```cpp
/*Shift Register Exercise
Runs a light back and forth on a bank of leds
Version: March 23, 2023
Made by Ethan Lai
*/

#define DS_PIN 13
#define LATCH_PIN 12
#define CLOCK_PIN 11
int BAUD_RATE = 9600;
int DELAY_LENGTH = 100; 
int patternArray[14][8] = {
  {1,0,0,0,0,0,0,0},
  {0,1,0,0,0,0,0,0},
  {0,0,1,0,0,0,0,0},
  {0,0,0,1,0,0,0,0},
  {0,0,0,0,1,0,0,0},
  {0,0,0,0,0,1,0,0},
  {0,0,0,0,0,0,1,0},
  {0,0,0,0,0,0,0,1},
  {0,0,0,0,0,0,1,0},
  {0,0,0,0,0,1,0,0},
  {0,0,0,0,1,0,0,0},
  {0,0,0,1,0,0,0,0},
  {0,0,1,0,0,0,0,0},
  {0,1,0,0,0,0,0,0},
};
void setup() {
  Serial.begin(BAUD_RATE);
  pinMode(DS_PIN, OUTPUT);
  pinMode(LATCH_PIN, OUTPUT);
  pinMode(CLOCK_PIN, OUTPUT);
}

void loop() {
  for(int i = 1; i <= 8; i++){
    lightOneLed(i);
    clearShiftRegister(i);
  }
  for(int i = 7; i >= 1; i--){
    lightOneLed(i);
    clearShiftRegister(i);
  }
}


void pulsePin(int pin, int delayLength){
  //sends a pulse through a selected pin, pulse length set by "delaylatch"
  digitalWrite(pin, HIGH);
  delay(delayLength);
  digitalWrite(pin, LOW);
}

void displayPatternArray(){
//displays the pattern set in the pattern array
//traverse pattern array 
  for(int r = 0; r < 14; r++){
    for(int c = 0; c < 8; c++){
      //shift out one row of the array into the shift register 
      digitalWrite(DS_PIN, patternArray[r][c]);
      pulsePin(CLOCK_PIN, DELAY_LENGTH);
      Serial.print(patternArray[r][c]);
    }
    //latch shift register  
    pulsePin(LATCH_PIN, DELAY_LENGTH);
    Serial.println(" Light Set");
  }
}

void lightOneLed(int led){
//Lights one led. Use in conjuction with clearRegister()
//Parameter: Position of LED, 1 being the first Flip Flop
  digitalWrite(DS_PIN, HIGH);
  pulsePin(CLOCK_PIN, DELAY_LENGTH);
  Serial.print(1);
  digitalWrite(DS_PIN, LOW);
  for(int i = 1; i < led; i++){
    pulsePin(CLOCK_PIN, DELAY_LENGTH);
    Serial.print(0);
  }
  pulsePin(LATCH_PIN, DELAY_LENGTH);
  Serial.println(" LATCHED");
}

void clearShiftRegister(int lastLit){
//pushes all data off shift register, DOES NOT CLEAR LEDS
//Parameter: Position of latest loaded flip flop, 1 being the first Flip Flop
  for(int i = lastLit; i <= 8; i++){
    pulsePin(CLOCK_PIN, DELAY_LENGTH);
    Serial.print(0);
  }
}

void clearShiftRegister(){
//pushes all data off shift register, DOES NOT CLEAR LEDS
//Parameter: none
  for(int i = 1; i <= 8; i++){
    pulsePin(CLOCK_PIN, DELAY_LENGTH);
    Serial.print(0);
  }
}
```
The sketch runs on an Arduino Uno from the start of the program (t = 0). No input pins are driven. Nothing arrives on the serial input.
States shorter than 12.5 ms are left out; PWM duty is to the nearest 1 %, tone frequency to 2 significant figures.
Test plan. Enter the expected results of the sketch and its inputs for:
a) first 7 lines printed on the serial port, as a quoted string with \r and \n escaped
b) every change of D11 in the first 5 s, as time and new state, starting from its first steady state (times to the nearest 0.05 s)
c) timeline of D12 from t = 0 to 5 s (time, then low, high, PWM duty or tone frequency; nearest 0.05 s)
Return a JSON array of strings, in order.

["\"1 LATCHED\\r\\n0000000010 LATCHED\\r\\n0000000100 LATCHED\\r\\n0000001000 LATCHED\\r\\n0000010000 LATCHED\\r\\n0000100000 LATCHED\\r\\n0001000000 LATCHED\\r\\n\"", "0 s high; 0.1 s low; 0.2 s high; 1.2 s low; 1.3 s high; 2.3 s low; 2.4 s high; 3.4 s low; 3.5 s high; 4.5 s low; 4.6 s high", "0 s low; 0.1 s high; 0.2 s low; 1.2 s high; 1.3 s low; 2.3 s high; 2.4 s low; 3.4 s high; 3.5 s low; 4.5 s high; 4.6 s low"]
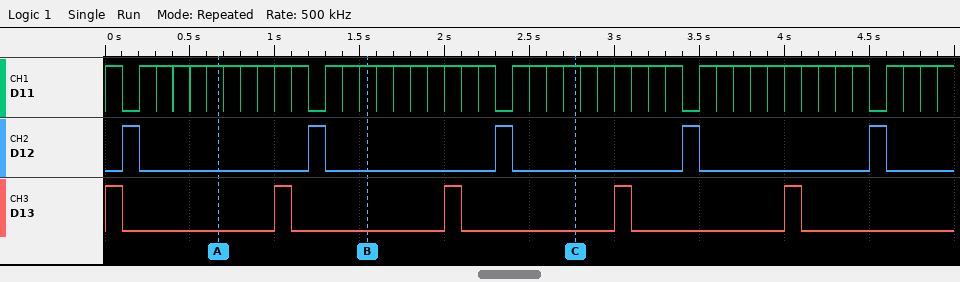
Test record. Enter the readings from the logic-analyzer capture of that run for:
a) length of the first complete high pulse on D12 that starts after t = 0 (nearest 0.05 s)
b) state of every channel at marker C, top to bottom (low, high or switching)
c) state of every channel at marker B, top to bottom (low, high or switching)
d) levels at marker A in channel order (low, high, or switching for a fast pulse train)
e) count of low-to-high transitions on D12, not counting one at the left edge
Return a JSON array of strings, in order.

["0.10 s", "D11 high, D12 low, D13 low", "D11 high, D12 low, D13 low", "D11 high, D12 low, D13 low", "5"]
